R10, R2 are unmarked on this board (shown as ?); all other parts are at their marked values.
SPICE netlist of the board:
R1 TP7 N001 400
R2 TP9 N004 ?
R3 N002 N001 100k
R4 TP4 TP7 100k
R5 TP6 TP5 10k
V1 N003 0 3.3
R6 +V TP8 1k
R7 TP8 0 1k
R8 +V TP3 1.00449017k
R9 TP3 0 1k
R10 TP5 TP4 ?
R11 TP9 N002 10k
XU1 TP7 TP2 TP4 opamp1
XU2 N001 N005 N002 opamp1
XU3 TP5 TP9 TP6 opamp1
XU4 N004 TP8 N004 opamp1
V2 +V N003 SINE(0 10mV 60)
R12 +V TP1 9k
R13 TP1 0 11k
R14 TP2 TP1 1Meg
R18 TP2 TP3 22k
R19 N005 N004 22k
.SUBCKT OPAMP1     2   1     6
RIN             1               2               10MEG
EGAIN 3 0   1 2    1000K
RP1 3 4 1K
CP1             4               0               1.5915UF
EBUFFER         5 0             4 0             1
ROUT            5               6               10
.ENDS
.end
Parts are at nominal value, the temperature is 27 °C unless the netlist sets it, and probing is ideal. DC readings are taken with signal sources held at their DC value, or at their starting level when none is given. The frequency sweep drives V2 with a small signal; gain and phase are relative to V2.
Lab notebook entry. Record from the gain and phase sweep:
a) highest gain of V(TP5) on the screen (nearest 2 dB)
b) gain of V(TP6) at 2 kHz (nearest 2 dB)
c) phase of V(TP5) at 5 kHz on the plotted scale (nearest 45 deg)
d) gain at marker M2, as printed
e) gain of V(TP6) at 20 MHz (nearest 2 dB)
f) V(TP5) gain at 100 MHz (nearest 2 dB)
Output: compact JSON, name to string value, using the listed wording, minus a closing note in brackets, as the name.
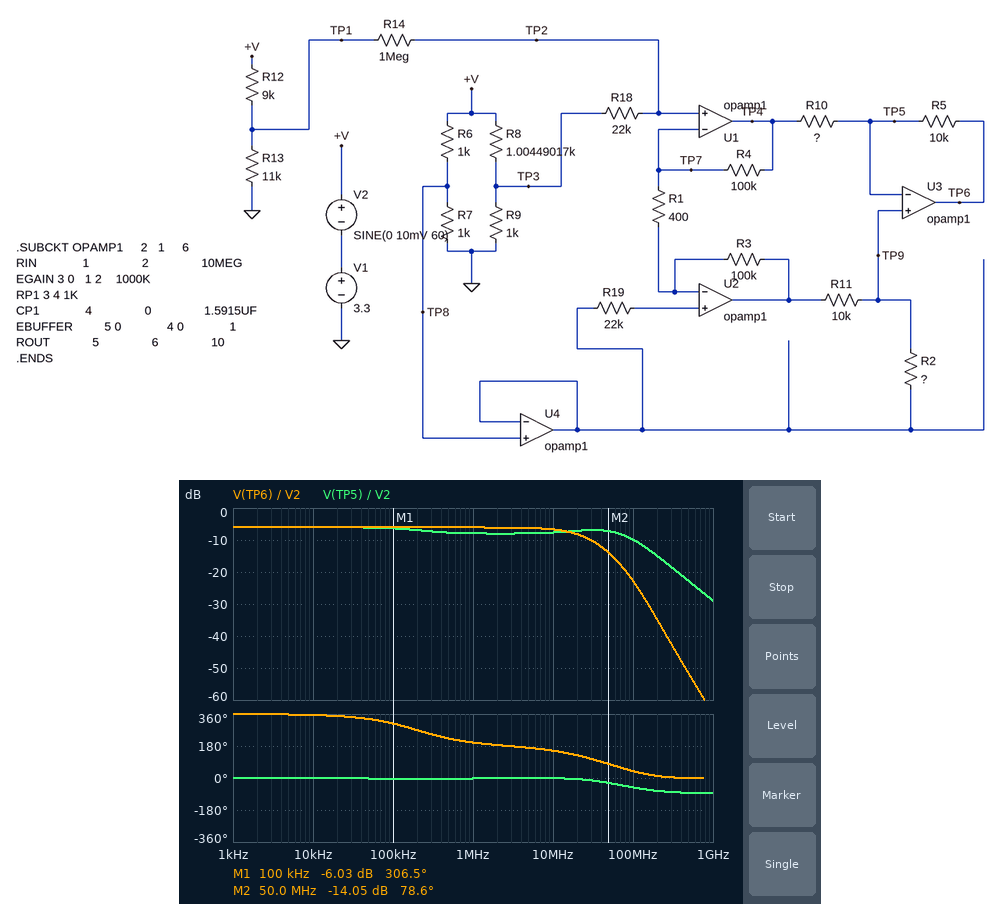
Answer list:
{"highest gain of V(TP5) on the screen": "-6 dB", "gain of V(TP6) at 2 kHz": "-6 dB", "phase of V(TP5) at 5 kHz on the plotted scale": "0 deg", "gain at marker M2, as printed": "-14.05 dB", "gain of V(TP6) at 20 MHz": "-8 dB", "V(TP5) gain at 100 MHz": "-10 dB"}
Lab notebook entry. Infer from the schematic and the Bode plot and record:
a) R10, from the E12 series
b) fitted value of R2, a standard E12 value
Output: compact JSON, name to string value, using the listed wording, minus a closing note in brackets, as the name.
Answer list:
{"R10, from the E12 series": "3.9 kΩ", "fitted value of R2, a standard E12 value": "6.8 kΩ"}
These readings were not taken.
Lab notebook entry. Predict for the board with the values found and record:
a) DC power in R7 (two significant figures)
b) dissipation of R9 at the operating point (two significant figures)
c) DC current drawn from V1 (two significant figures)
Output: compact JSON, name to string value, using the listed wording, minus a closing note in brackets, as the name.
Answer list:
{"DC power in R7": "2.7 mW", "dissipation of R9 at the operating point": "2.7 mW", "DC current drawn from V1": "3.5 mA"}
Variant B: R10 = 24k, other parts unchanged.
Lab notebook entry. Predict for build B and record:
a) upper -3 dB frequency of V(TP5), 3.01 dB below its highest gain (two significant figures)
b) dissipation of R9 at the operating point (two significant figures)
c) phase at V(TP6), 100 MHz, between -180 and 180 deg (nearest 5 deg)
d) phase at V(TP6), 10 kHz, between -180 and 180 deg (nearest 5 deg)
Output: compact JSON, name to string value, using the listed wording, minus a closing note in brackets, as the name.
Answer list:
{"upper -3 dB frequency of V(TP5), 3.01 dB below its highest gain": "31 MHz", "dissipation of R9 at the operating point": "2.7 mW", "phase at V(TP6), 100 MHz, between -180 and 180 deg": "-105 deg", "phase at V(TP6), 10 kHz, between -180 and 180 deg": "0 deg"}
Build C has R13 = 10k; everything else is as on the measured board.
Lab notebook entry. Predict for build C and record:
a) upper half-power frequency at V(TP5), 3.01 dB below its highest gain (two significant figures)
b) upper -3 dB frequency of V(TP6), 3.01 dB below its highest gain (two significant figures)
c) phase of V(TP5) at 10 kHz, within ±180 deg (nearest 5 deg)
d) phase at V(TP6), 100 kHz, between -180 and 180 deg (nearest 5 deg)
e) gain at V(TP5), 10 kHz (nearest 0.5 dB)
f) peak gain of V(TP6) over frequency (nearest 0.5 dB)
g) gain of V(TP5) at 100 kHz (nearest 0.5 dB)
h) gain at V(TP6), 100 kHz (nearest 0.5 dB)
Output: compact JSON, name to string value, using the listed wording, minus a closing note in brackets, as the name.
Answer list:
{"upper half-power frequency at V(TP5), 3.01 dB below its highest gain": "70 MHz", "upper -3 dB frequency of V(TP6), 3.01 dB below its highest gain": "270 kHz", "phase of V(TP5) at 10 kHz, within ±180 deg": "0 deg", "phase at V(TP6), 100 kHz, between -180 and 180 deg": "-40 deg", "gain at V(TP5), 10 kHz": "-5.0 dB", "peak gain of V(TP6) over frequency": "0 dB", "gain of V(TP5) at 100 kHz": "-5.5 dB", "gain at V(TP6), 100 kHz": "-0.5 dB"}
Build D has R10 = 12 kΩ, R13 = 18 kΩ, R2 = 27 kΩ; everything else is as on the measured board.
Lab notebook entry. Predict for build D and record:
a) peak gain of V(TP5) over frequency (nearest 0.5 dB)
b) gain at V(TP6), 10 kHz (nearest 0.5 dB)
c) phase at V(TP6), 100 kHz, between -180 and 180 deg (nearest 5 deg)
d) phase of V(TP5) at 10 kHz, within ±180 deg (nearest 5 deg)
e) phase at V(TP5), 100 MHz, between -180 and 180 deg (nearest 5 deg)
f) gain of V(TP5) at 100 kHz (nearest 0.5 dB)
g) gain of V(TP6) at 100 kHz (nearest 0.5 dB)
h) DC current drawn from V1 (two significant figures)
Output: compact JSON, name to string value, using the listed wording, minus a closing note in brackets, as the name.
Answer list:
{"peak gain of V(TP5) over frequency": "-10.0 dB", "gain at V(TP6), 10 kHz": "-1.0 dB", "phase at V(TP6), 100 kHz, between -180 and 180 deg": "155 deg", "phase of V(TP5) at 10 kHz, within ±180 deg": "20 deg", "phase at V(TP5), 100 MHz, between -180 and 180 deg": "-55 deg", "gain of V(TP5) at 100 kHz": "-16.5 dB", "gain of V(TP6) at 100 kHz": "-2.0 dB", "DC current drawn from V1": "3.4 mA"}
